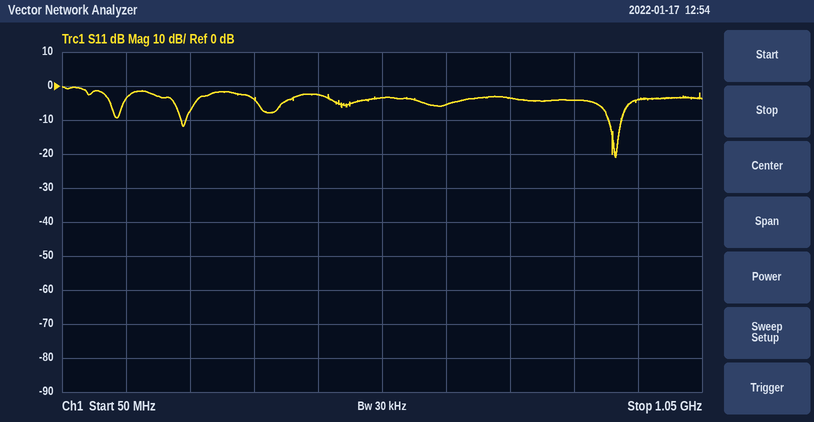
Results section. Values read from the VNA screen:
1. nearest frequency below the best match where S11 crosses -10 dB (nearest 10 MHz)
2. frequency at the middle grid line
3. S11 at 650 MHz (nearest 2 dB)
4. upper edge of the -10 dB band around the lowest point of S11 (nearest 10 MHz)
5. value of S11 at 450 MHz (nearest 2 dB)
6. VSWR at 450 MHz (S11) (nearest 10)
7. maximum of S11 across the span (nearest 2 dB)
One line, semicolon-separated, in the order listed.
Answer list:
900 MHz; 550 MHz; -6 dB; 920 MHz; -2 dB; 10; 0 dB
